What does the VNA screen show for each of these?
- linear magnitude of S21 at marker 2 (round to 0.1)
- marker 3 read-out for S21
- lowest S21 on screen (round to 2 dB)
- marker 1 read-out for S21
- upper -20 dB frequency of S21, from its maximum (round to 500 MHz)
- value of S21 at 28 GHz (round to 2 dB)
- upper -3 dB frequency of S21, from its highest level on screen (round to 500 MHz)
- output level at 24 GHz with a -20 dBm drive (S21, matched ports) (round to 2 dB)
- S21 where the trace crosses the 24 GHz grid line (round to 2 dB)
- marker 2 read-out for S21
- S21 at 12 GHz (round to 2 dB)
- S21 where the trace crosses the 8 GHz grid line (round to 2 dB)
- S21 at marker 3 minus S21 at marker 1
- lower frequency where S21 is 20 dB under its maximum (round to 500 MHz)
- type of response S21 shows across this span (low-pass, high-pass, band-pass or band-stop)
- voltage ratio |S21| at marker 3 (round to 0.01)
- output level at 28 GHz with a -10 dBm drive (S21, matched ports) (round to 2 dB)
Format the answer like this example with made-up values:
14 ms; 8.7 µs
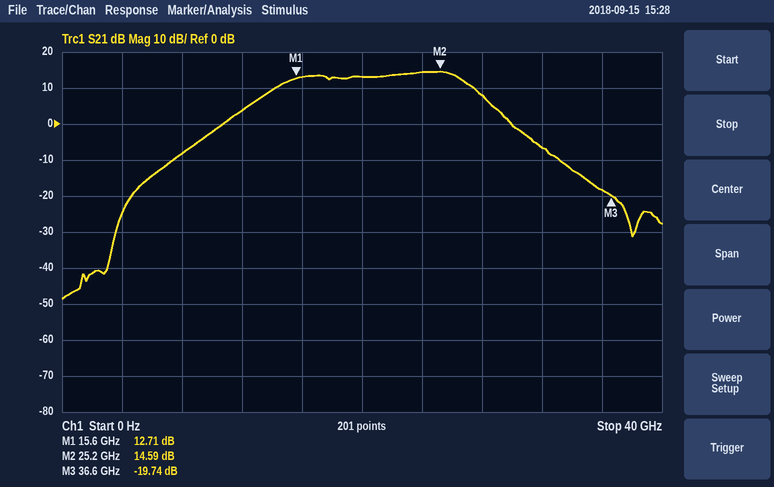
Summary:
5.4; -19.74 dB; -48 dB; 12.71 dB; 31.5 GHz; 8 dB; 27.0 GHz; -6 dBm; 14 dB; 14.59 dB; 4 dB; -8 dB; -32.45 dB; 9.0 GHz; band-pass; 0.10; -2 dBm
